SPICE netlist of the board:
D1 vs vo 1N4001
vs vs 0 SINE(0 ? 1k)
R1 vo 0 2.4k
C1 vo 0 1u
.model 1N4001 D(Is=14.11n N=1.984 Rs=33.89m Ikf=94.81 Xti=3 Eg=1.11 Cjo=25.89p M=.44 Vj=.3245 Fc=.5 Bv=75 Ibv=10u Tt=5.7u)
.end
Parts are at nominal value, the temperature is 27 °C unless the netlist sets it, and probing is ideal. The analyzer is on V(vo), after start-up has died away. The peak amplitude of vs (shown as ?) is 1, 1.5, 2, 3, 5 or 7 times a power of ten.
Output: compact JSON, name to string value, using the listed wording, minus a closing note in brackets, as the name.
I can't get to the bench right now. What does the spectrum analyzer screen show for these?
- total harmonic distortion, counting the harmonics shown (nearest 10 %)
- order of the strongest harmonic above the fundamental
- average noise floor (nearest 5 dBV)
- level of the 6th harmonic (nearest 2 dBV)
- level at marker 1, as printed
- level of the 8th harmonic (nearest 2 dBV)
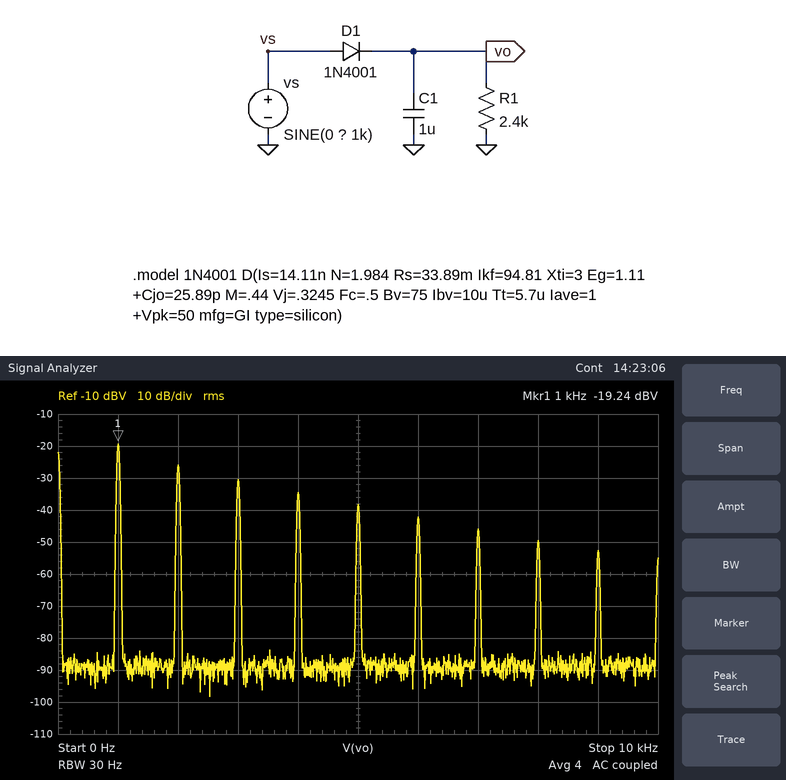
{"total harmonic distortion, counting the harmonics shown": "60 %", "order of the strongest harmonic above the fundamental": "2", "average noise floor": "-90 dBV", "level of the 6th harmonic": "-42 dBV", "level at marker 1, as printed": "-19.24 dBV", "level of the 8th harmonic": "-50 dBV"}
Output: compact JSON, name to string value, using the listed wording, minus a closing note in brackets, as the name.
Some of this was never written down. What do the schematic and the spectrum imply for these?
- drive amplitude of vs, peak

{"drive amplitude of vs, peak": "2 V"}
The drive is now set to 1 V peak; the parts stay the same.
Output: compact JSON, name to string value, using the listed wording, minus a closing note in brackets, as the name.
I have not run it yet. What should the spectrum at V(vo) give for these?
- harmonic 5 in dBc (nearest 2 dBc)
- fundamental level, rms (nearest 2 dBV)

{"harmonic 5 in dBc": "-20 dBc", "fundamental level, rms": "-30 dBV"}
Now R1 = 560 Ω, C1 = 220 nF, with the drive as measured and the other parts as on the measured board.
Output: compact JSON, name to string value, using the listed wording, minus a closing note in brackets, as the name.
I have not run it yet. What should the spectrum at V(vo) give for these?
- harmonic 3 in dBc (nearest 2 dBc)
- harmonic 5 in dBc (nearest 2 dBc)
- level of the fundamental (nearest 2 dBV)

{"harmonic 3 in dBc": "-16 dBc", "harmonic 5 in dBc": "-28 dBc", "level of the fundamental": "-8 dBV"}
